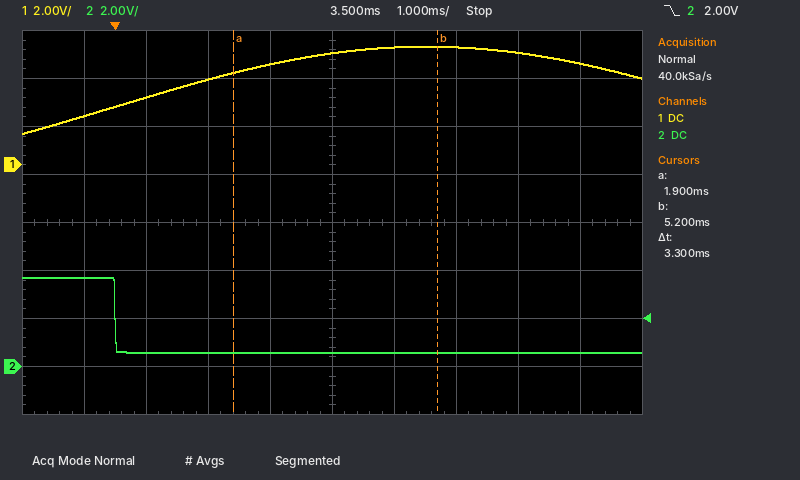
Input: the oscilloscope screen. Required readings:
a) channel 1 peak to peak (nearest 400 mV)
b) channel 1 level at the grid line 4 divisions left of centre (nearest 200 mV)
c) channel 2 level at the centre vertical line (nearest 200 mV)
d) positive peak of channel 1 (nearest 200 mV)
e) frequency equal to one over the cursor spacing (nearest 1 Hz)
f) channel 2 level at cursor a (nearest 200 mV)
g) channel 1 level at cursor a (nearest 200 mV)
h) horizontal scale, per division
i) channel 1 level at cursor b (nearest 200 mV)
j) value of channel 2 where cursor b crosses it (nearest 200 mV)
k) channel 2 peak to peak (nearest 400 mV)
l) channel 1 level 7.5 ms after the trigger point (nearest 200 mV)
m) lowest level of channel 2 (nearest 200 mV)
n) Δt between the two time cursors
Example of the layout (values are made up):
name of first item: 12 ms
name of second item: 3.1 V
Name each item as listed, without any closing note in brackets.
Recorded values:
channel 1 peak to peak: 3.6 V
channel 1 level at the grid line 4 divisions left of centre: 2.0 V
channel 2 level at the centre vertical line: 600 mV
positive peak of channel 1: 5.0 V
frequency equal to one over the cursor spacing: 303 Hz
channel 2 level at cursor a: 600 mV
channel 1 level at cursor a: 3.8 V
horizontal scale, per division: 1 ms
channel 1 level at cursor b: 5.0 V
value of channel 2 where cursor b crosses it: 600 mV
channel 2 peak to peak: 3.2 V
channel 1 level 7.5 ms after the trigger point: 4.2 V
lowest level of channel 2: 600 mV
Δt between the two time cursors: 3.3 ms
